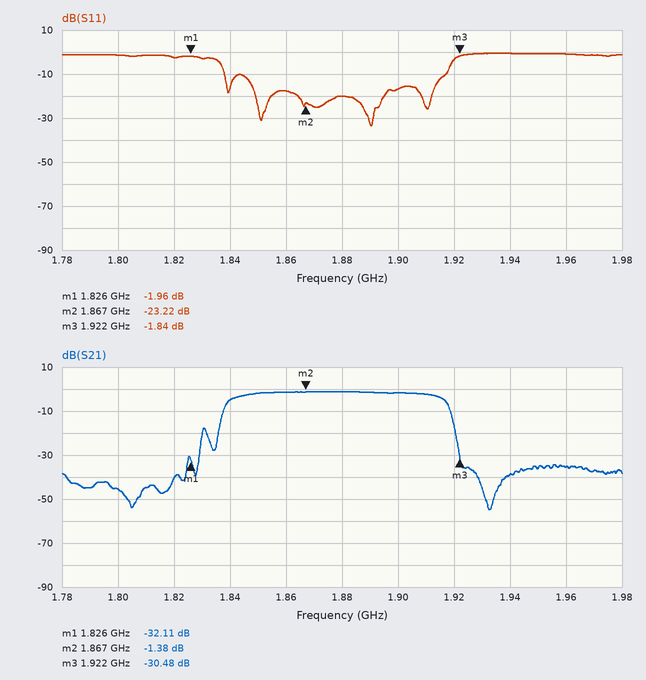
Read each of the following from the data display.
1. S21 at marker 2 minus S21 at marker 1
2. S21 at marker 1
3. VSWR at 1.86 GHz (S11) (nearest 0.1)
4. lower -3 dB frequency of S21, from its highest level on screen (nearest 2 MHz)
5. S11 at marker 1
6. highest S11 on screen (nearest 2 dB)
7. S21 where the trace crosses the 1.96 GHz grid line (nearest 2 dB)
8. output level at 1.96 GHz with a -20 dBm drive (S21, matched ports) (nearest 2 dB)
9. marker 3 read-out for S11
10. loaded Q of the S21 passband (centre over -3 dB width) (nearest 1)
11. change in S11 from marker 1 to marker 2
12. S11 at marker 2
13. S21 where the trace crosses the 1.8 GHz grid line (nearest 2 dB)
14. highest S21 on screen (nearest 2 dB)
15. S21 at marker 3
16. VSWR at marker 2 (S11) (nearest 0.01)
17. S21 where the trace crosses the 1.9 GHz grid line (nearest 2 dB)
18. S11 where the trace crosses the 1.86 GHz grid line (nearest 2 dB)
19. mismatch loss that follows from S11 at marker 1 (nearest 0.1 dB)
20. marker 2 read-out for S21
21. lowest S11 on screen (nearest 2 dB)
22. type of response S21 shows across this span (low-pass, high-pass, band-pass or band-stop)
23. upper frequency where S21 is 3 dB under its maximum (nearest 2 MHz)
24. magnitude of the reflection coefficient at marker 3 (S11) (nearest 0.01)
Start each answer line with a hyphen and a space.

- 30.73 dB
- -32.11 dB
- 1.3
- 1.842 GHz
- -1.96 dB
- 0 dB
- -36 dB
- -56 dBm
- -1.84 dB
- 25
- -21.26 dB
- -23.22 dB
- -46 dB
- -2 dB
- -30.48 dB
- 1.15
- -2 dB
- -18 dB
- 4.4 dB
- -1.38 dB
- -34 dB
- band-pass
- 1.916 GHz
- 0.81
